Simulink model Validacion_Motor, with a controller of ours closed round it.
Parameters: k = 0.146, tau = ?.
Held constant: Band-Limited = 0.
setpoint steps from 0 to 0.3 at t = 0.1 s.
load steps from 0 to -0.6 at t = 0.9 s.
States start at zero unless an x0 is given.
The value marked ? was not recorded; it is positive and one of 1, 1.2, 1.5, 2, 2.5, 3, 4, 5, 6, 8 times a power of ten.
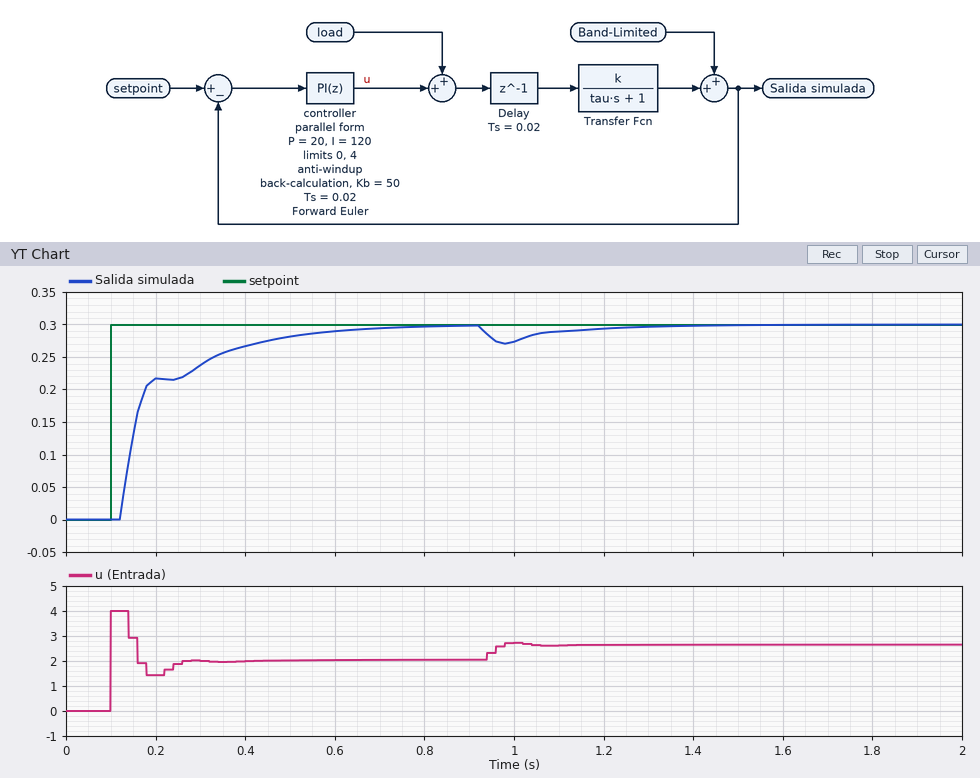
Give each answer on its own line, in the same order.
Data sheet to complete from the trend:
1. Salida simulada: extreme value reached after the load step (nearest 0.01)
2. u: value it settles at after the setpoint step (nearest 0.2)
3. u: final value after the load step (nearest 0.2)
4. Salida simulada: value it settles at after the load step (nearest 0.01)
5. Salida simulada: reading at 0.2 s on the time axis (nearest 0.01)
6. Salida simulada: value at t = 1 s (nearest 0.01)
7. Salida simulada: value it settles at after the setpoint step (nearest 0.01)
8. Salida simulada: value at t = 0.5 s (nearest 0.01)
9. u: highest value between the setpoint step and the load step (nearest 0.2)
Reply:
0.27
2.0
2.6
0.30
0.22
0.27
0.30
0.28
4.0
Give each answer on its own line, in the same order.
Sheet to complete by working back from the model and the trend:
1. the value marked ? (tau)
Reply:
0.12
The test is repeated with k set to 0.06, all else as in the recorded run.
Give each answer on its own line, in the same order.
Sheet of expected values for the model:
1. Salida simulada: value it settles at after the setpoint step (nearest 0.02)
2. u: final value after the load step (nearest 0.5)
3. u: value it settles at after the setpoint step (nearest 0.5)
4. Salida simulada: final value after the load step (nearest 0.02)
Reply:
0.24
4.0
4.0
0.20
